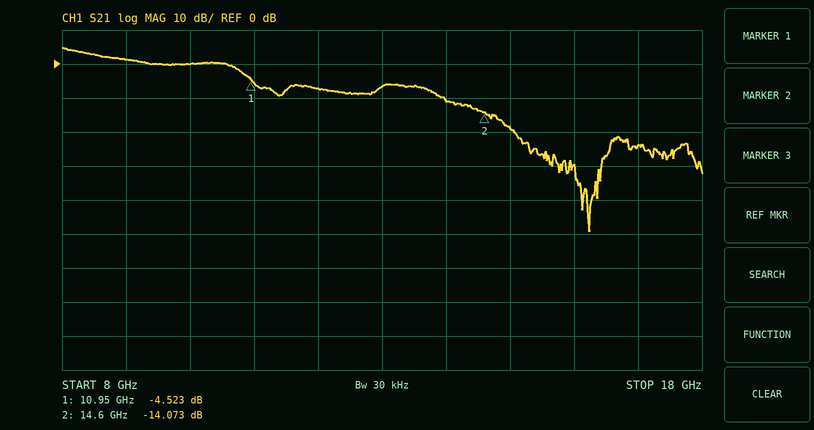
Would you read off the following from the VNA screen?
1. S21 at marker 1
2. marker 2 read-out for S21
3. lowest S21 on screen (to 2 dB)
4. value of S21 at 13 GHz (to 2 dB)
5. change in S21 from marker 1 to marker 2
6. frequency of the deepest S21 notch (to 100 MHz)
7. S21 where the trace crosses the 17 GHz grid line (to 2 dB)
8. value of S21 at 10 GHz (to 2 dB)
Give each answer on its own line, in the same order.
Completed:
-4.523 dB
-14.073 dB
-50 dB
-6 dB
-9.550 dB
16.2 GHz
-24 dB
0 dB
